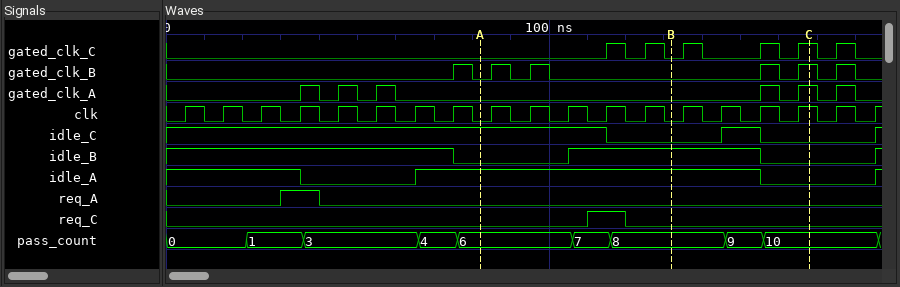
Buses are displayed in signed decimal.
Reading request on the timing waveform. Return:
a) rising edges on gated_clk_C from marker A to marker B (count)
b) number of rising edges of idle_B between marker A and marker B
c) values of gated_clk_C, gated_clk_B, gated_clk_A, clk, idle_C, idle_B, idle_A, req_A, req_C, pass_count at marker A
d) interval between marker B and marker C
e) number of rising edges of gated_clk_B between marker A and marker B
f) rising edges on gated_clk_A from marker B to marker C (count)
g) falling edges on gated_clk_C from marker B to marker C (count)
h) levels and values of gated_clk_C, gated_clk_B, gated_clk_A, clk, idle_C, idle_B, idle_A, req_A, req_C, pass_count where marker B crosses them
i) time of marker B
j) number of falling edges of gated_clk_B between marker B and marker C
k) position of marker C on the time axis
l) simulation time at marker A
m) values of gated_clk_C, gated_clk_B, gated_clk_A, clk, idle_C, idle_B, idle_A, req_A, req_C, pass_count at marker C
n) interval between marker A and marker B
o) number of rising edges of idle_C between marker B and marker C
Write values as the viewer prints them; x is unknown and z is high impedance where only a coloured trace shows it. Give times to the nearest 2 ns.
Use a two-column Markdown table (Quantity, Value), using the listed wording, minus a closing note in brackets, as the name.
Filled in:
| Quantity | Value |
|---|---|
| rising edges on gated_clk_C from marker A to marker B | 2 |
| number of rising edges of idle_B between marker A and marker B | 1 |
| values of gated_clk_C, gated_clk_B, gated_clk_A, clk, idle_C, idle_B, idle_A, req_A, req_C, pass_count at marker A | gated_clk_C=0, gated_clk_B=0, gated_clk_A=0, clk=0, idle_C=1, idle_B=0, idle_A=1, req_A=0, req_C=0, pass_count=6 |
| interval between marker B and marker C | 36 ns |
| number of rising edges of gated_clk_B between marker A and marker B | 2 |
| rising edges on gated_clk_A from marker B to marker C | 2 |
| falling edges on gated_clk_C from marker B to marker C | 2 |
| levels and values of gated_clk_C, gated_clk_B, gated_clk_A, clk, idle_C, idle_B, idle_A, req_A, req_C, pass_count where marker B crosses them | gated_clk_C=0, gated_clk_B=0, gated_clk_A=0, clk=0, idle_C=0, idle_B=1, idle_A=1, req_A=0, req_C=0, pass_count=8 |
| time of marker B | 132 ns |
| number of falling edges of gated_clk_B between marker B and marker C | 1 |
| position of marker C on the time axis | 168 ns |
| simulation time at marker A | 82 ns |
| values of gated_clk_C, gated_clk_B, gated_clk_A, clk, idle_C, idle_B, idle_A, req_A, req_C, pass_count at marker C | gated_clk_C=1, gated_clk_B=1, gated_clk_A=1, clk=1, idle_C=0, idle_B=0, idle_A=0, req_A=0, req_C=0, pass_count=10 |
| interval between marker A and marker B | 50 ns |
| number of rising edges of idle_C between marker B and marker C | 1 |
